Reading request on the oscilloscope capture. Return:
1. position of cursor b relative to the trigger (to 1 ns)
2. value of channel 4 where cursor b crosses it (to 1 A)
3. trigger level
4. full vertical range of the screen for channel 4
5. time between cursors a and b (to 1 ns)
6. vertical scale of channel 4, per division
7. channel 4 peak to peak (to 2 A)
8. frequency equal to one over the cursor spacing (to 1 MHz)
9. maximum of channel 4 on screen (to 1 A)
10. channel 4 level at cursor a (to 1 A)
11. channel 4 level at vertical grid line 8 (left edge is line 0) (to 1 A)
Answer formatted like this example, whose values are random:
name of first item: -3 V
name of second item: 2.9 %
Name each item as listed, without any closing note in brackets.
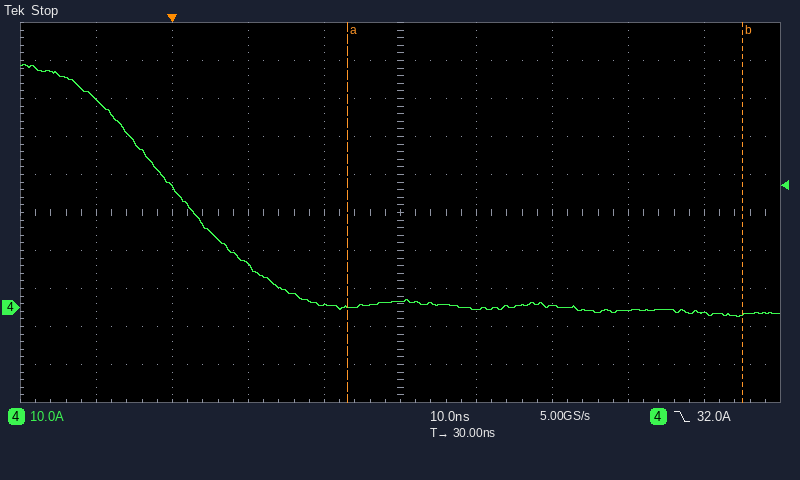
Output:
position of cursor b relative to the trigger: +75 ns
value of channel 4 where cursor b crosses it: -2 A
trigger level: 32.0 A
full vertical range of the screen for channel 4: 100 A
time between cursors a and b: 52 ns
vertical scale of channel 4, per division: 10 A
channel 4 peak to peak: 66 A
frequency equal to one over the cursor spacing: 19 MHz
maximum of channel 4 on screen: 64 A
channel 4 level at cursor a: 0 A
channel 4 level at vertical grid line 8 (left edge is line 0): -1 A
